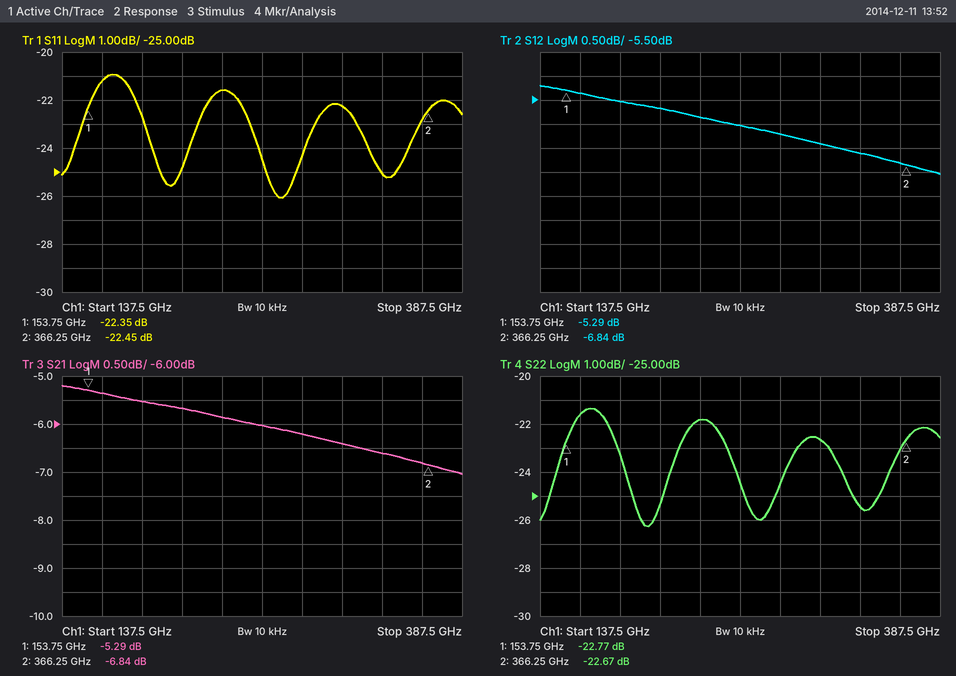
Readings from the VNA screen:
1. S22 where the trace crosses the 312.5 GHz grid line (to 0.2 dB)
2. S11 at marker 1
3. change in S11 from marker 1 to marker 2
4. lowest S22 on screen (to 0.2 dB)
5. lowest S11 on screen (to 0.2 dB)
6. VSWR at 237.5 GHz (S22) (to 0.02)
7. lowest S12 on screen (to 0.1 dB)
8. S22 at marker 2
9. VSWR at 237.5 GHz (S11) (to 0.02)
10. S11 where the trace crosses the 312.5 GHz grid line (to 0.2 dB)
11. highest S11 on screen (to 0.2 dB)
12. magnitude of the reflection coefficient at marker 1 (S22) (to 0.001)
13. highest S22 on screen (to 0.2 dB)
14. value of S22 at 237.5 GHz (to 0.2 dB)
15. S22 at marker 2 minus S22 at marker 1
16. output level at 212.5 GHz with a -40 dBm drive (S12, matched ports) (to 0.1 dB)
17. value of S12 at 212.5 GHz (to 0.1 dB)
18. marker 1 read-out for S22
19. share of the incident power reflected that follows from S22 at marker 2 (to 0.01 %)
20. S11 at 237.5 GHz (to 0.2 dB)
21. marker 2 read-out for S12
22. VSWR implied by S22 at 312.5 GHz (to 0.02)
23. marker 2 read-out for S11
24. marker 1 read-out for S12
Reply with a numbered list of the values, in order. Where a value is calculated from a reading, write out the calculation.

1. -22.6 dB
2. -22.35 dB
3. -22.45 − (-22.35) = -0.10 dB
4. -26.2 dB
5. -26.0 dB
6. |Γ| = 10^(-21.8/20) = 0.0813; VSWR = (1 + 0.0813)/(1 − 0.0813) ≈ 1.18
7. -7.0 dB
8. -22.67 dB
9. |Γ| = 10^(-21.6/20) = 0.0832; VSWR = (1 + 0.0832)/(1 − 0.0832) ≈ 1.18
10. -22.2 dB
11. -21.0 dB
12. 10^(-22.77/20) ≈ 0.073
13. -21.4 dB
14. -21.8 dB
15. -22.67 − (-22.77) = 0.10 dB
16. -40 dBm + (-5.7 dB) = -45.7 dBm
17. -5.7 dB
18. -22.77 dB
19. 10^(-22.67/10) ≈ 0.54 %
20. -21.6 dB
21. -6.84 dB
22. |Γ| = 10^(-22.6/20) = 0.0741; VSWR = (1 + 0.0741)/(1 − 0.0741) ≈ 1.16
23. -22.45 dB
24. -5.29 dB
